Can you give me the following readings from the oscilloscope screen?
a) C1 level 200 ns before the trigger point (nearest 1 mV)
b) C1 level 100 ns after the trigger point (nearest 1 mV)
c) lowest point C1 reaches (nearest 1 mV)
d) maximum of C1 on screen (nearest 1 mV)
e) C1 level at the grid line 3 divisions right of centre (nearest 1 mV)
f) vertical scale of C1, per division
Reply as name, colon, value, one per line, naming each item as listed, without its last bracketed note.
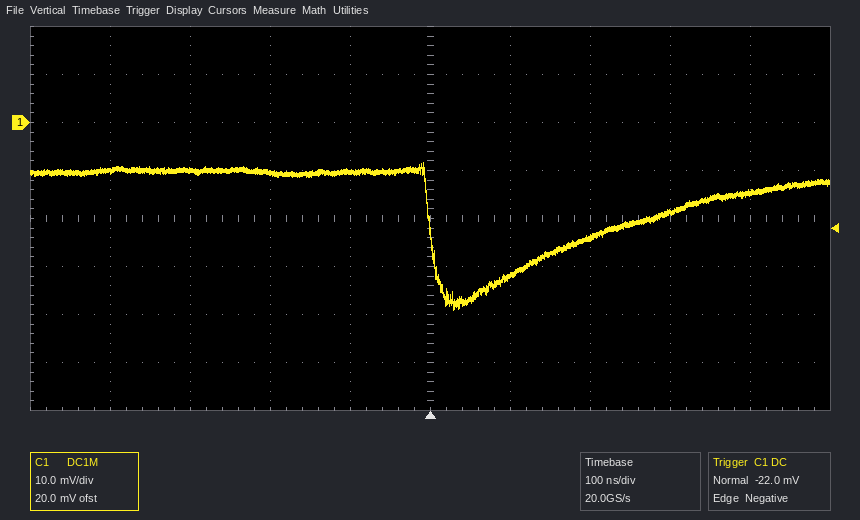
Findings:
C1 level 200 ns before the trigger point: -10 mV
C1 level 100 ns after the trigger point: -32 mV
lowest point C1 reaches: -39 mV
maximum of C1 on screen: -8 mV
C1 level at the grid line 3 divisions right of centre: -19 mV
vertical scale of C1, per division: 10 mV
